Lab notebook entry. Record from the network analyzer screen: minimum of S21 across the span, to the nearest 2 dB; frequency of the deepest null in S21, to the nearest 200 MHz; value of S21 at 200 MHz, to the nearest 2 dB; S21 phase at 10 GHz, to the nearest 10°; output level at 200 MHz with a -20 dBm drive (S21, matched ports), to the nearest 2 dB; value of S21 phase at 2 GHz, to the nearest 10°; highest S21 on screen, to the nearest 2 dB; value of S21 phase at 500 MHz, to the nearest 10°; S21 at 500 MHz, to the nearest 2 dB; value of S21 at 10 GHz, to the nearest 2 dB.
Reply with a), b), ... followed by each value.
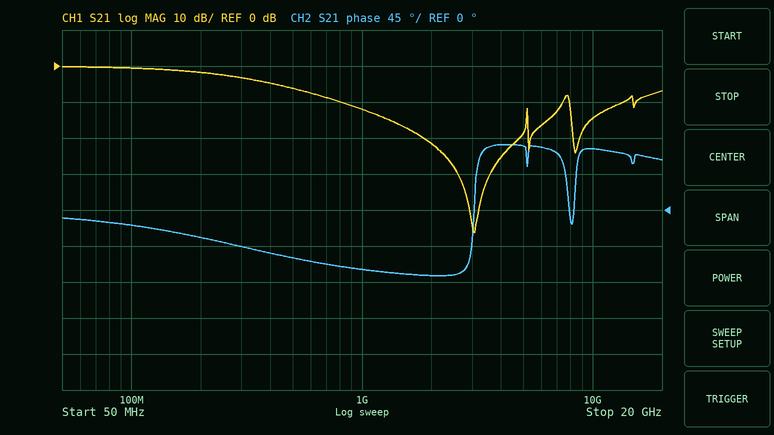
a) -46 dB
b) 3.0 GHz
c) -2 dB
d) 80°
e) -22 dBm
f) -80°
g) 0 dB
h) -60°
i) -6 dB
j) -14 dB
